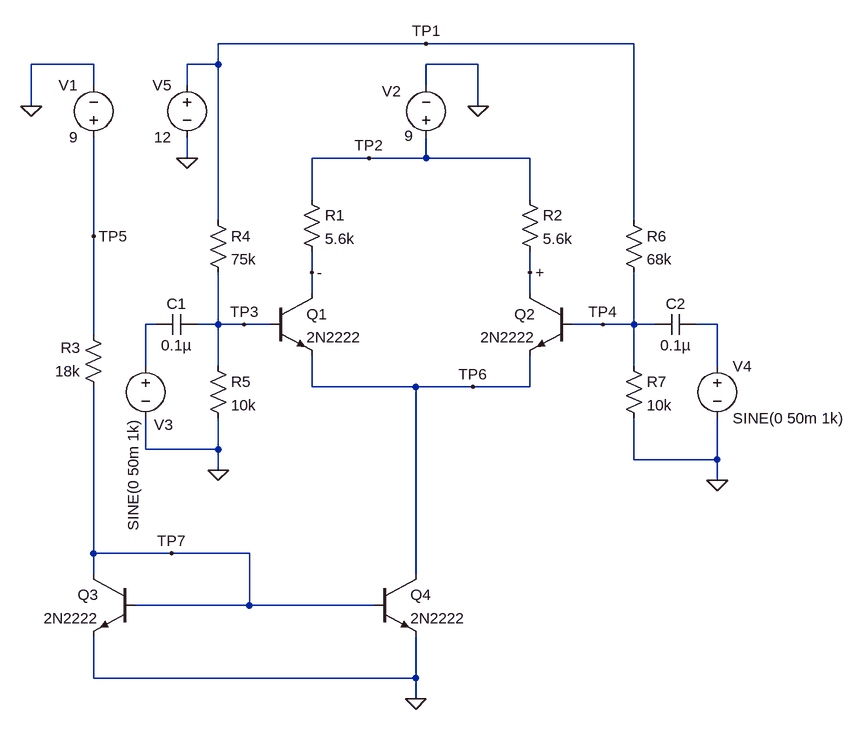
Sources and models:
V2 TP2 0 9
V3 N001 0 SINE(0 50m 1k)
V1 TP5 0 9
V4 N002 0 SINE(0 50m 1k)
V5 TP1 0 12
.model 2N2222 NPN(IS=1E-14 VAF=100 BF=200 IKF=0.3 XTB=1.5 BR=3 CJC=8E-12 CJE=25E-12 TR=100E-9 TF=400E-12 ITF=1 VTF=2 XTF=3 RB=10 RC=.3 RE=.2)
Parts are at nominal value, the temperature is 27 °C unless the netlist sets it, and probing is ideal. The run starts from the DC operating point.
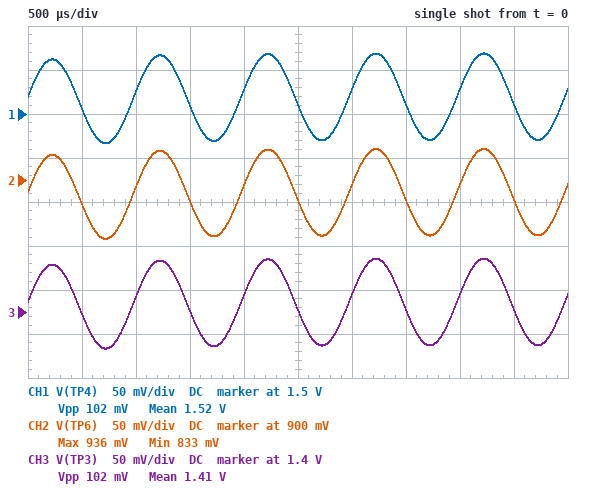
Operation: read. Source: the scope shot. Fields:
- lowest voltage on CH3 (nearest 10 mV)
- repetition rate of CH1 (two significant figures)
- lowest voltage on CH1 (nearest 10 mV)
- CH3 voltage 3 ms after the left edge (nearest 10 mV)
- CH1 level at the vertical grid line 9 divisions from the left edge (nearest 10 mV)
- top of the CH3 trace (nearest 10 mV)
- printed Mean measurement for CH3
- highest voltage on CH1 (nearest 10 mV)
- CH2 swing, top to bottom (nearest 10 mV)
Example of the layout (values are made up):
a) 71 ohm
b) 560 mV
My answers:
a) 1.36 V
b) 1.0 kHz
c) 1.47 V
d) 1.42 V
e) 1.51 V
f) 1.46 V
g) 1.41 V
h) 1.57 V
i) 100 mV
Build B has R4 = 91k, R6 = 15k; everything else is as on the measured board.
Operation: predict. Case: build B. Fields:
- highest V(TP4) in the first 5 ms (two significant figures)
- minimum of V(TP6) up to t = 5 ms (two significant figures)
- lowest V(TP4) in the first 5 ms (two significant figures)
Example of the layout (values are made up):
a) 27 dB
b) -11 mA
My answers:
a) 4.8 V
b) 4.1 V
c) 4.7 V
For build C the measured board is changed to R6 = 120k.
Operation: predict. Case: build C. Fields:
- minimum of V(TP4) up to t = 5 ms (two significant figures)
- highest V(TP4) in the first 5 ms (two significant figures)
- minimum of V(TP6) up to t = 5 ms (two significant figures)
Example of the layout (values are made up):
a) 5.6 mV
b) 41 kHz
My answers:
a) 870 mV
b) 970 mV
c) 710 mV
